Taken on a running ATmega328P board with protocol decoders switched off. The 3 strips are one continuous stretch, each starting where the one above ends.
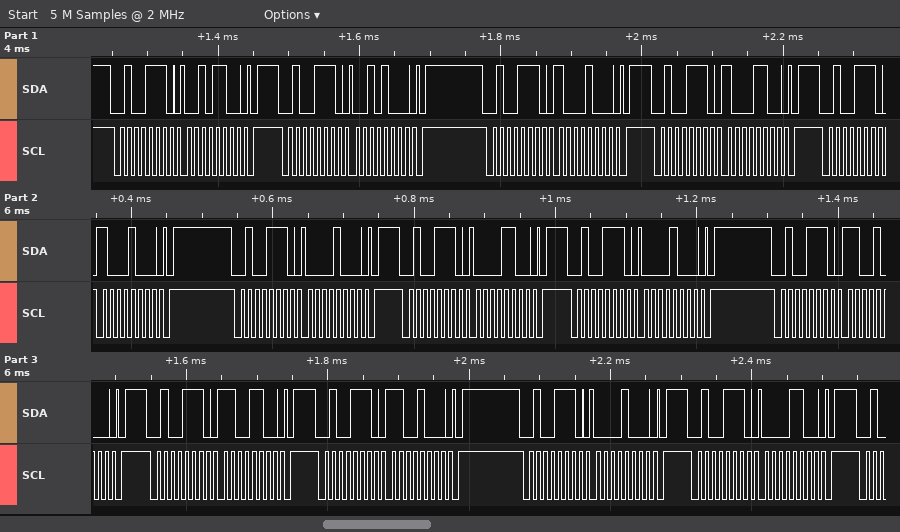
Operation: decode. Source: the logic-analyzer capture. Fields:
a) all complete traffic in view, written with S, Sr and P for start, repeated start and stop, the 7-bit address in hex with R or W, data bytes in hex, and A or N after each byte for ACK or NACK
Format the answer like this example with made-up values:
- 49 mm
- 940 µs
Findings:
- S 27W A 2C A P S 27W A 28 A P S 27W A 88 A P S 27W A 8C A P S 27W A 88 A P S 27W A 08 A P S 27W A 0C A P S 27W A 08 A P S 27W A C8 A P S 27W A CC A P S 27W A C8 A P S 27W A 08 A P S 27W A 0C A P
